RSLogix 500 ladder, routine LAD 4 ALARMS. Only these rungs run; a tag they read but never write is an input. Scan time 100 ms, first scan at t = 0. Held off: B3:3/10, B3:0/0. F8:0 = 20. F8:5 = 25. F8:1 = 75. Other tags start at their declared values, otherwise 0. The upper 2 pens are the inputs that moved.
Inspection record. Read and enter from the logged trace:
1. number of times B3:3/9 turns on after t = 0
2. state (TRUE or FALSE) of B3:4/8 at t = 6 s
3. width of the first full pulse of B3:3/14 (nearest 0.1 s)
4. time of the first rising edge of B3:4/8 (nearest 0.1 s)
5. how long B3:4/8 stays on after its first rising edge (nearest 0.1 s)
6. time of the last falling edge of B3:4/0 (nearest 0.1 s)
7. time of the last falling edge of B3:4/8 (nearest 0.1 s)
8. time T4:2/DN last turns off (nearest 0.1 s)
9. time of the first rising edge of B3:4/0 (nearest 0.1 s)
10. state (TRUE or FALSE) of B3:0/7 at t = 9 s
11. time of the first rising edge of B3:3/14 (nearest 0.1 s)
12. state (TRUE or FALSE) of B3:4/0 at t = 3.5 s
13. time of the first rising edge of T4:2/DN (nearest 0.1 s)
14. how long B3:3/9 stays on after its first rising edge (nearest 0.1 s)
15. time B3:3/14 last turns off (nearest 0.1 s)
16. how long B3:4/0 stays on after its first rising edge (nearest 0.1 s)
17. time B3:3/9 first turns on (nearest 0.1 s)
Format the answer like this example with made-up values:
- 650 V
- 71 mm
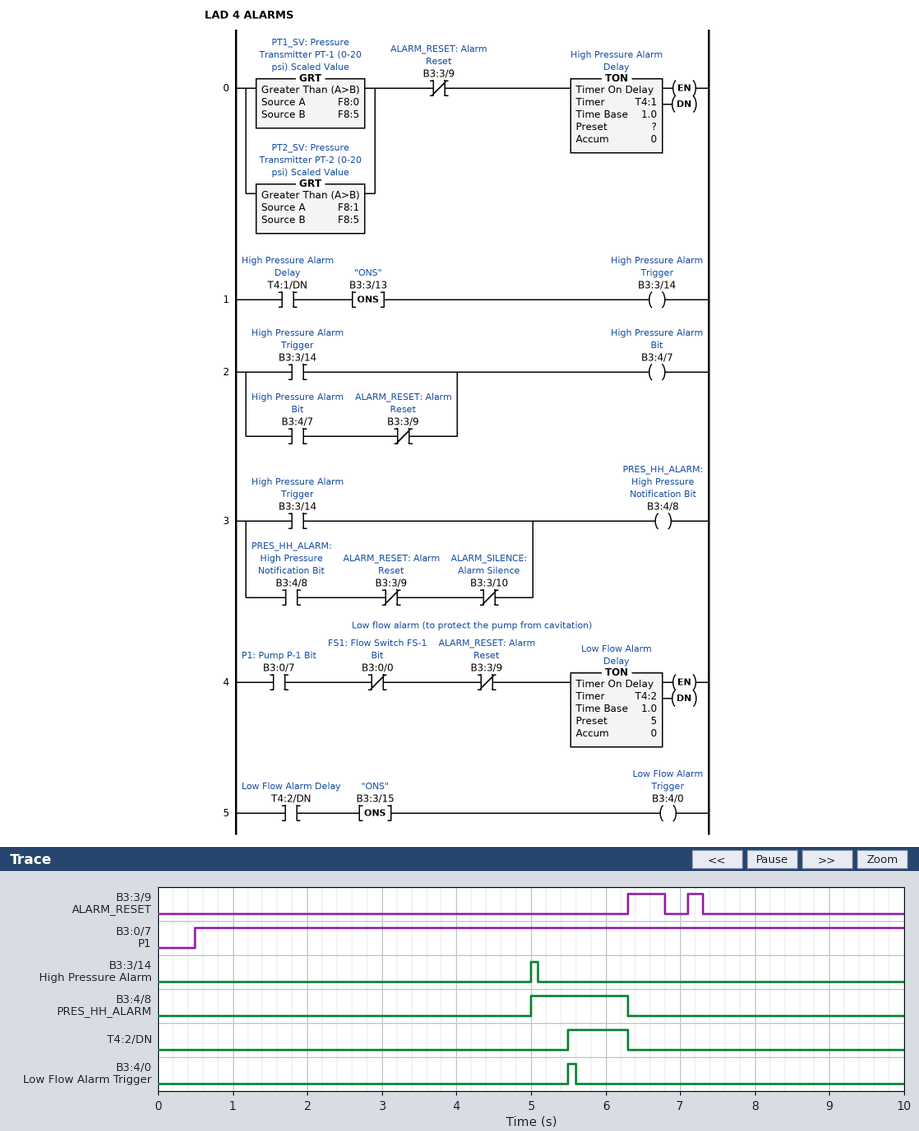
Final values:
- 2
- TRUE
- 0.1 s
- 5.0 s
- 1.3 s
- 5.6 s
- 6.3 s
- 6.3 s
- 5.5 s
- TRUE
- 5.0 s
- FALSE
- 5.5 s
- 0.5 s
- 5.1 s
- 0.1 s
- 6.3 s
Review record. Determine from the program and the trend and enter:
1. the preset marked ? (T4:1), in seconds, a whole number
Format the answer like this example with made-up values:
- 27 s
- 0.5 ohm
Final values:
- 5 s
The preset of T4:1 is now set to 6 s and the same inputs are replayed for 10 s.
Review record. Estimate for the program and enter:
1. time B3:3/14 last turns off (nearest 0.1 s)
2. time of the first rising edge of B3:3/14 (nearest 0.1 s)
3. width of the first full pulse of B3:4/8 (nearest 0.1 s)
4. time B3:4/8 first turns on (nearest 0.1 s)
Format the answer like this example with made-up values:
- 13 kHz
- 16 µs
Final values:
- 6.1 s
- 6.0 s
- 0.3 s
- 6.0 s
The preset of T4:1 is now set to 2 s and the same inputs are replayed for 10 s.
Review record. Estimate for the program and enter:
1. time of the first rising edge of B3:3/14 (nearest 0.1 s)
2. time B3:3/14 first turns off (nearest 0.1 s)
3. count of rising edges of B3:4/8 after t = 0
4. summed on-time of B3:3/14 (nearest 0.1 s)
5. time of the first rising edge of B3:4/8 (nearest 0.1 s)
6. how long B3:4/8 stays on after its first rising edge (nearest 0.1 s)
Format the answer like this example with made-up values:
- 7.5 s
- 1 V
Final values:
- 2.0 s
- 2.1 s
- 2
- 0.2 s
- 2.0 s
- 4.3 s
